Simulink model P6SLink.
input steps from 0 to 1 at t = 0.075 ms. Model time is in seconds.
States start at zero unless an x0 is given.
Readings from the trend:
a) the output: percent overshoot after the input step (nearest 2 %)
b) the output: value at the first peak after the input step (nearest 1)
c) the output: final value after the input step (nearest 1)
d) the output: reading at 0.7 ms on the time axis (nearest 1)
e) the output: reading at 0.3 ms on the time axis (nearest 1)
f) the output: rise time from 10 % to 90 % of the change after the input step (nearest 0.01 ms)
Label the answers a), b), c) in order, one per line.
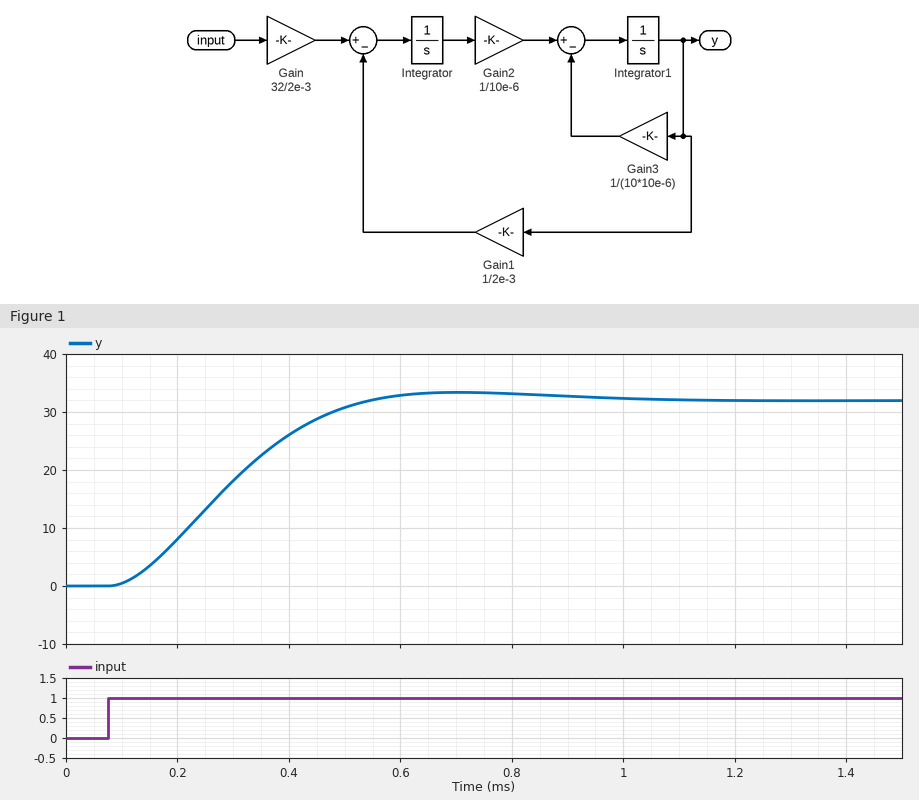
a) 4 %
b) 33
c) 32
d) 33
e) 18
f) 0.30 ms
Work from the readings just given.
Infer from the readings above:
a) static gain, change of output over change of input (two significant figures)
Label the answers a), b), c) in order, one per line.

a) 32
